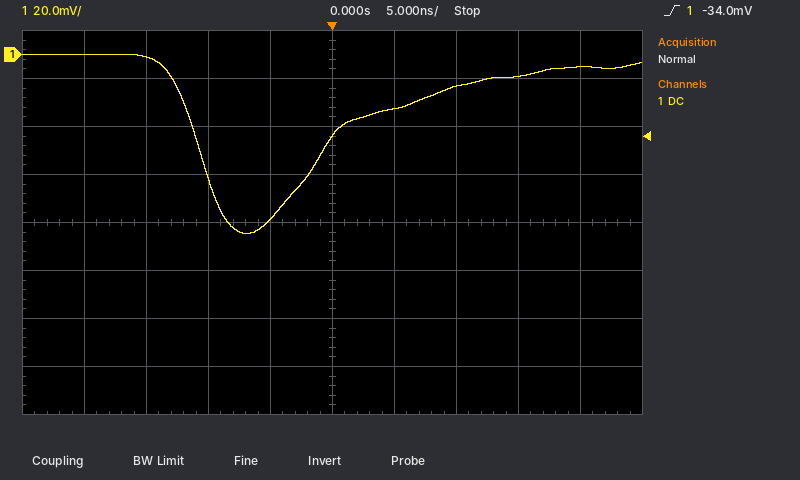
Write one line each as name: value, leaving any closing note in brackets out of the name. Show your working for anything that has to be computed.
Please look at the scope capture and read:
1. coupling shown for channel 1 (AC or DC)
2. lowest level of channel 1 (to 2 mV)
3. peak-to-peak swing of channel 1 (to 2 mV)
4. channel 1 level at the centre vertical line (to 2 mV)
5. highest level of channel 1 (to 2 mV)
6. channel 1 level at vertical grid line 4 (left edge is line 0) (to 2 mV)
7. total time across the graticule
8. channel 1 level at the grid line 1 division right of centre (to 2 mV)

coupling shown for channel 1: DC
lowest level of channel 1: -74 mV
peak-to-peak swing of channel 1: 0 mV − (-74 mV) = 74 mV
channel 1 level at the centre vertical line: -34 mV
highest level of channel 1: 0 mV
channel 1 level at vertical grid line 4 (left edge is line 0): -68 mV
total time across the graticule: 50 ns
channel 1 level at the grid line 1 division right of centre: -22 mV
